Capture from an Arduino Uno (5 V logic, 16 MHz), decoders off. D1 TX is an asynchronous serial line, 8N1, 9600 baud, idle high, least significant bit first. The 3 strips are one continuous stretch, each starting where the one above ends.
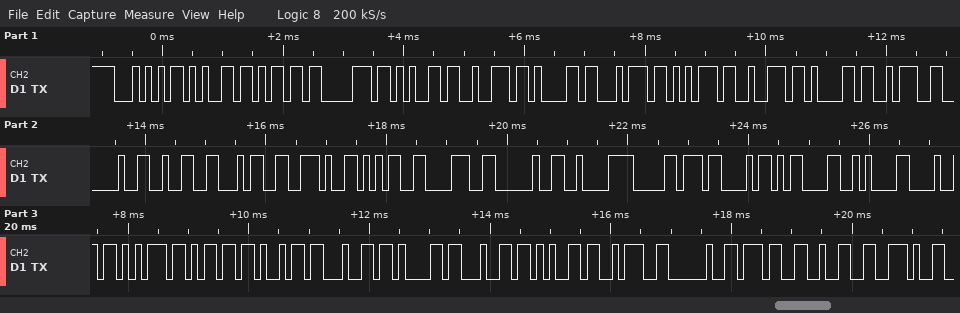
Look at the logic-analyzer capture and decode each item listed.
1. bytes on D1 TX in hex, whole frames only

54 65 6D 70 65 72 61 74 75 72 61 3A 20 32 34 2E 35 38 20 C2 B0 43 0D 0A 48 75 6D 69 64 61 64 65 3A 20 37 32 2E
